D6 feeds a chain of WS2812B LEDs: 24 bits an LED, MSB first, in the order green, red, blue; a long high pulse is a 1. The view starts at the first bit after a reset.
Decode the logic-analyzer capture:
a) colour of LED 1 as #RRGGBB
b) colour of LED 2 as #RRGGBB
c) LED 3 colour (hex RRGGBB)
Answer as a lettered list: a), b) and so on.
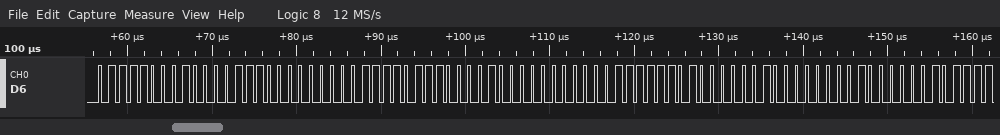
a) #877800
b) #847B00
c) #817E00
